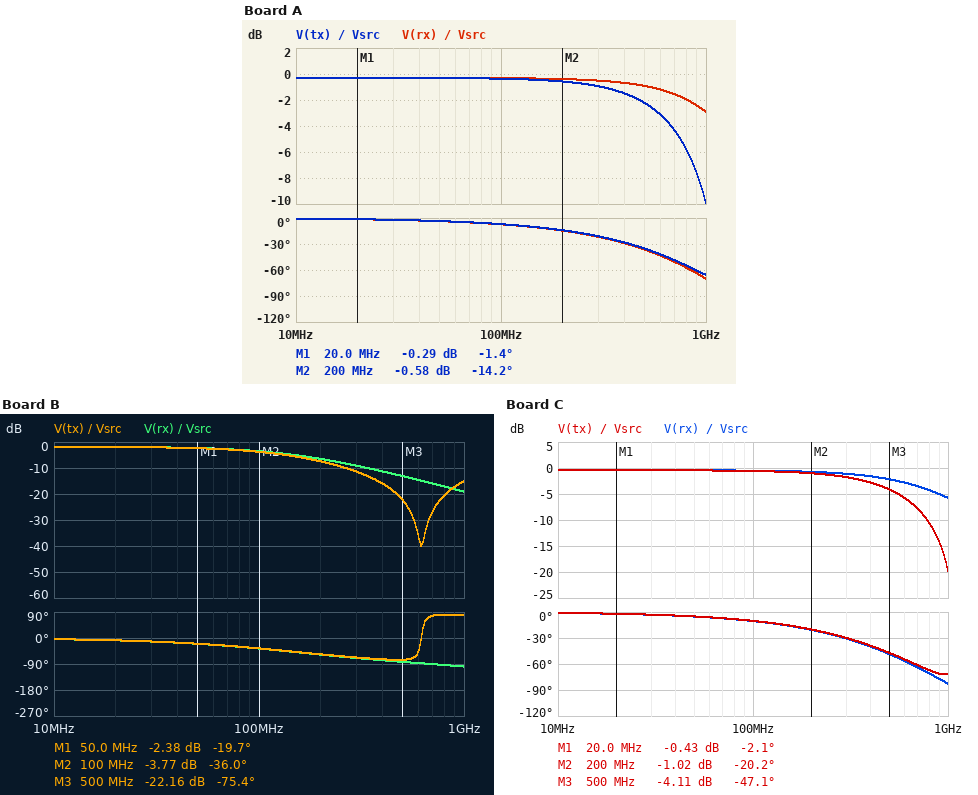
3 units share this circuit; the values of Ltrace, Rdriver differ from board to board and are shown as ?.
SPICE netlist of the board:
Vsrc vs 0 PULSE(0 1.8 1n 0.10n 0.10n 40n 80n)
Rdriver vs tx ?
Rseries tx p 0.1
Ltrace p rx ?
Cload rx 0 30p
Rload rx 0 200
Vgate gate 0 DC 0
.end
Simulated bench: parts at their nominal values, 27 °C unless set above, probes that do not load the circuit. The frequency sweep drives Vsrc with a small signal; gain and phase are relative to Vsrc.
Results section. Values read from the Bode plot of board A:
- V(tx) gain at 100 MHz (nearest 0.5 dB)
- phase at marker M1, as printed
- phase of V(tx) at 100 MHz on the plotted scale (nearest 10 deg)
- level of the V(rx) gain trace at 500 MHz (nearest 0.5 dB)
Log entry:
-0.5 dB
-1.4 deg
-10 deg
-1.0 dB
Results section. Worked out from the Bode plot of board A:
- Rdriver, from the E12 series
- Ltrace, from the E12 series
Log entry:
6.8 Ω
470 pH
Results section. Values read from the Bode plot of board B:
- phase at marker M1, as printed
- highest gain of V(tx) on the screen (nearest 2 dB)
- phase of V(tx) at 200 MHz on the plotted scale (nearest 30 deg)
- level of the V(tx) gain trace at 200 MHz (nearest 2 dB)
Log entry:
-19.7 deg
-2 dB
-60 deg
-8 dB
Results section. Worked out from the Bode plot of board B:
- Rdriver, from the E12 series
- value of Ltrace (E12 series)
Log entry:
47 Ω
2.2 nH
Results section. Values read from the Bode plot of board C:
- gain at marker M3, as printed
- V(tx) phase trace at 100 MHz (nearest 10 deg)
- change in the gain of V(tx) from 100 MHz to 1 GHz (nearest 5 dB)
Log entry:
-4.11 dB
-10 deg
-20 dB
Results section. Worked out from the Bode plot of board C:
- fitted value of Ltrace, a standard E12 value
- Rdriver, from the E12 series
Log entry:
680 pH
10 Ω
